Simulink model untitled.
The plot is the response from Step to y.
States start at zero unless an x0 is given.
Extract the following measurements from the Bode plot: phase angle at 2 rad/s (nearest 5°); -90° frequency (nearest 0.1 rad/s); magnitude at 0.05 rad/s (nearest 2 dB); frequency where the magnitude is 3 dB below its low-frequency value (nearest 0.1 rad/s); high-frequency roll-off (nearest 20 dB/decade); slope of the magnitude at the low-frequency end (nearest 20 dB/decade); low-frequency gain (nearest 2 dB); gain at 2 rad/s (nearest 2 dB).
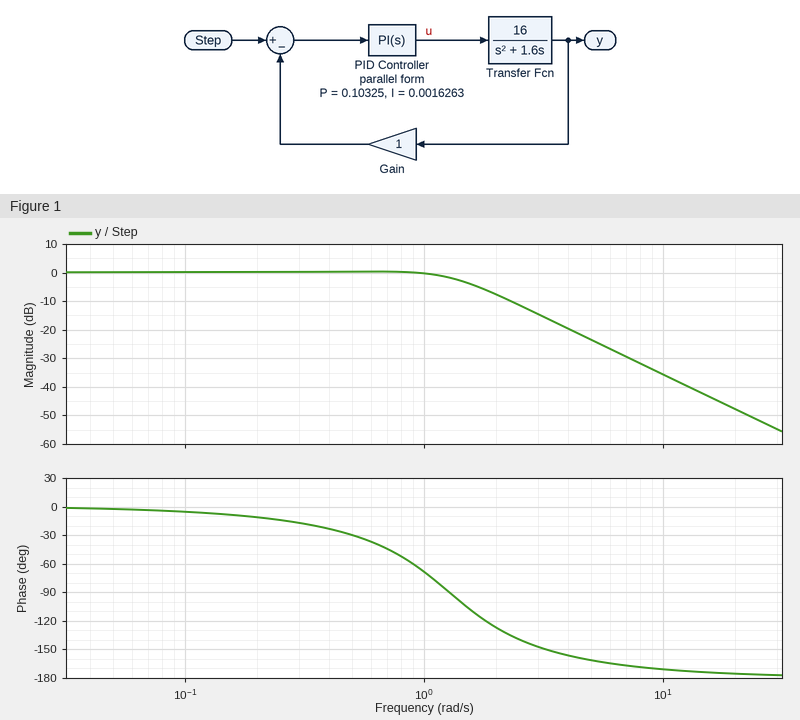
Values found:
-125°
1.3 rad/s
0 dB
1.4 rad/s
-40 dB/decade
0 dB/decade
0 dB
-8 dB
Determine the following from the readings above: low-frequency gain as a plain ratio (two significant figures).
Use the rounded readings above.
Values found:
1.0
